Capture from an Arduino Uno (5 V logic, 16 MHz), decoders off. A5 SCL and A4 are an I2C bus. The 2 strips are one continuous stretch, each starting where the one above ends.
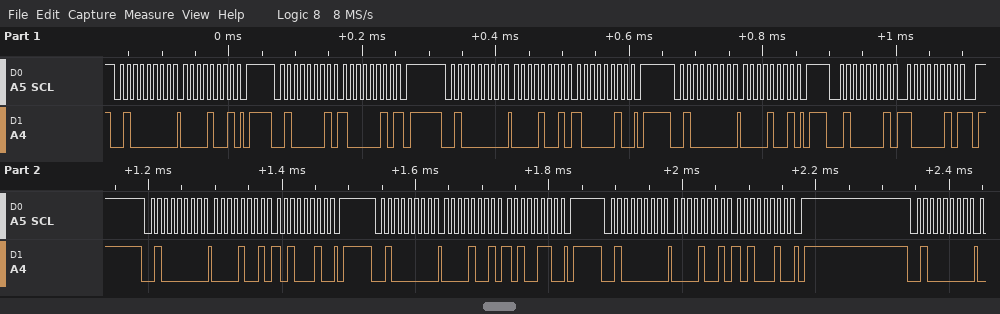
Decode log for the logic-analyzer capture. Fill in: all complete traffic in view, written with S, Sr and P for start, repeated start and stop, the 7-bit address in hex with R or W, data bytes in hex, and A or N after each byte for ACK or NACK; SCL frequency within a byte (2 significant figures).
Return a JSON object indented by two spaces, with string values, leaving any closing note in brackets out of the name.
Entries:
{
  "all complete traffic in view, written with S, Sr and P for start, repeated start and stop, the 7-bit address in hex with R or W, data bytes in hex, and A or N after each byte for ACK or NACK": "S 20W A 09 A P S 20R A 82 N P S 20W A 09 A 82 A P S 20W A 09 A P S 20R A 82 N P S 20W A 09 A A2 A P S 20W A 09 A A6 A P S 20W A 09 A A2 A P S 20W A",
  "SCL frequency within a byte": "100 kHz"
}
